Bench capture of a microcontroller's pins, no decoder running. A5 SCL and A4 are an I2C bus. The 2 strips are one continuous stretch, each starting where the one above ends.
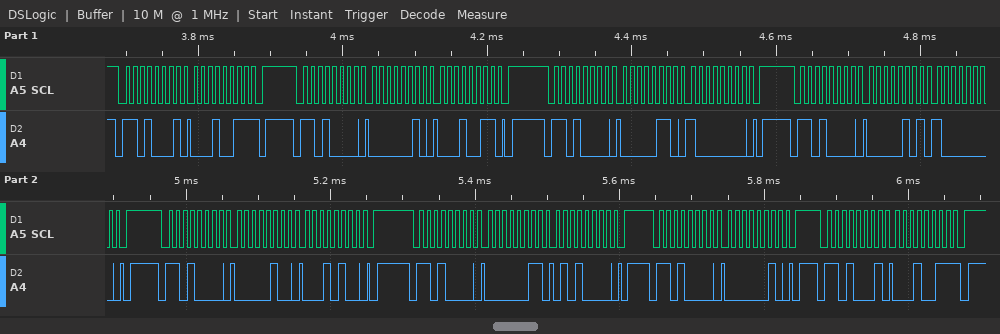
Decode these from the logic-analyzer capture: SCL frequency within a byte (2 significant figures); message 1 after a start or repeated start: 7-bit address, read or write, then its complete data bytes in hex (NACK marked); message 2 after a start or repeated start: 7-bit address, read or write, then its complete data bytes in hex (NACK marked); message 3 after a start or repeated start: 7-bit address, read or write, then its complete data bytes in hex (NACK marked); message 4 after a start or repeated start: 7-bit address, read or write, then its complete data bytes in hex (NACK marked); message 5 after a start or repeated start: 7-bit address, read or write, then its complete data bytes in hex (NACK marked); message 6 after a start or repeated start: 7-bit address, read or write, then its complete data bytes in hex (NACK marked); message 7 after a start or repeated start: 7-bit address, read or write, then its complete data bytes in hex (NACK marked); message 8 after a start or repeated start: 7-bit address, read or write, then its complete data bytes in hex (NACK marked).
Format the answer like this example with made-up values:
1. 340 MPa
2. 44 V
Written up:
1. 100 kHz
2. 0x68 read: 13 NACK
3. 0x68 write: 02 13
4. 0x68 write: 06 80
5. 0x68 write: 05 80
6. 0x68 write: 04 14
7. 0x68 write: 03 50
8. 0x68 write: 02
9. 0x68 read: 13 NACK
